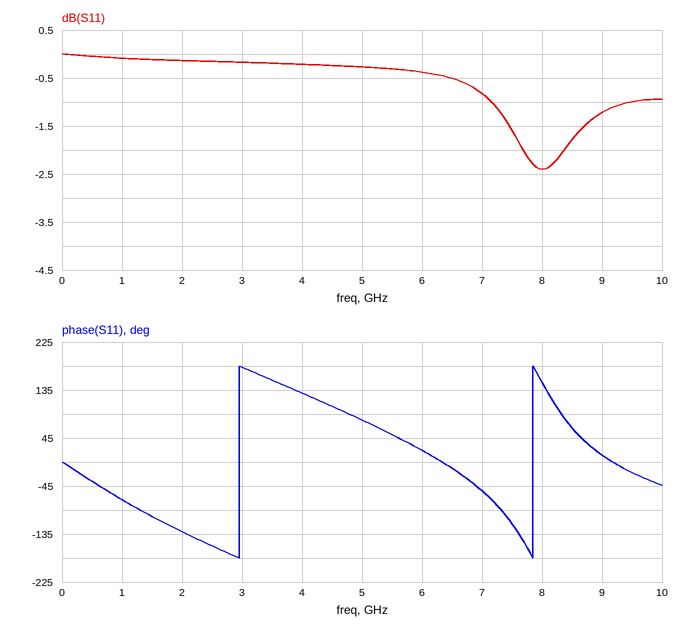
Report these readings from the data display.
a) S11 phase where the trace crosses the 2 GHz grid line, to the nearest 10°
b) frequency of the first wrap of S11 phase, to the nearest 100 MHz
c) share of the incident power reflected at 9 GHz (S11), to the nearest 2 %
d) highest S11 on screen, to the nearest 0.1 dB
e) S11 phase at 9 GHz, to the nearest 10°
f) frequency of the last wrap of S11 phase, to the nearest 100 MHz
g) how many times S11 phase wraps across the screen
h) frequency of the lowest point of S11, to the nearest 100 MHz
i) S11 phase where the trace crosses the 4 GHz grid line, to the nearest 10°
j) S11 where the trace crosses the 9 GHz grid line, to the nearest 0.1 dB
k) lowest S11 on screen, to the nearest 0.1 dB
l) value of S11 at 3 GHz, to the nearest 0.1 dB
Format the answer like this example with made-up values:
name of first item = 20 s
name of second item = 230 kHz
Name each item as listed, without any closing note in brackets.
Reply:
S11 phase where the trace crosses the 2 GHz grid line, to the nearest 10° = -130°
frequency of the first wrap of S11 phase, to the nearest 100 MHz = 3.0 GHz
share of the incident power reflected at 9 GHz (S11), to the nearest 2 % = 76 %
highest S11 on screen, to the nearest 0.1 dB = 0.0 dB
S11 phase at 9 GHz, to the nearest 10° = 10°
frequency of the last wrap of S11 phase, to the nearest 100 MHz = 7.8 GHz
how many times S11 phase wraps across the screen = 2
frequency of the lowest point of S11, to the nearest 100 MHz = 8.0 GHz
S11 phase where the trace crosses the 4 GHz grid line, to the nearest 10° = 130°
S11 where the trace crosses the 9 GHz grid line, to the nearest 0.1 dB = -1.2 dB
lowest S11 on screen, to the nearest 0.1 dB = -2.4 dB
value of S11 at 3 GHz, to the nearest 0.1 dB = -0.2 dB
